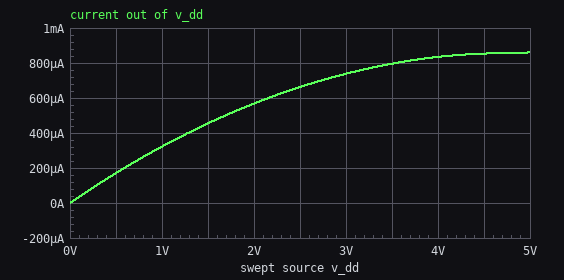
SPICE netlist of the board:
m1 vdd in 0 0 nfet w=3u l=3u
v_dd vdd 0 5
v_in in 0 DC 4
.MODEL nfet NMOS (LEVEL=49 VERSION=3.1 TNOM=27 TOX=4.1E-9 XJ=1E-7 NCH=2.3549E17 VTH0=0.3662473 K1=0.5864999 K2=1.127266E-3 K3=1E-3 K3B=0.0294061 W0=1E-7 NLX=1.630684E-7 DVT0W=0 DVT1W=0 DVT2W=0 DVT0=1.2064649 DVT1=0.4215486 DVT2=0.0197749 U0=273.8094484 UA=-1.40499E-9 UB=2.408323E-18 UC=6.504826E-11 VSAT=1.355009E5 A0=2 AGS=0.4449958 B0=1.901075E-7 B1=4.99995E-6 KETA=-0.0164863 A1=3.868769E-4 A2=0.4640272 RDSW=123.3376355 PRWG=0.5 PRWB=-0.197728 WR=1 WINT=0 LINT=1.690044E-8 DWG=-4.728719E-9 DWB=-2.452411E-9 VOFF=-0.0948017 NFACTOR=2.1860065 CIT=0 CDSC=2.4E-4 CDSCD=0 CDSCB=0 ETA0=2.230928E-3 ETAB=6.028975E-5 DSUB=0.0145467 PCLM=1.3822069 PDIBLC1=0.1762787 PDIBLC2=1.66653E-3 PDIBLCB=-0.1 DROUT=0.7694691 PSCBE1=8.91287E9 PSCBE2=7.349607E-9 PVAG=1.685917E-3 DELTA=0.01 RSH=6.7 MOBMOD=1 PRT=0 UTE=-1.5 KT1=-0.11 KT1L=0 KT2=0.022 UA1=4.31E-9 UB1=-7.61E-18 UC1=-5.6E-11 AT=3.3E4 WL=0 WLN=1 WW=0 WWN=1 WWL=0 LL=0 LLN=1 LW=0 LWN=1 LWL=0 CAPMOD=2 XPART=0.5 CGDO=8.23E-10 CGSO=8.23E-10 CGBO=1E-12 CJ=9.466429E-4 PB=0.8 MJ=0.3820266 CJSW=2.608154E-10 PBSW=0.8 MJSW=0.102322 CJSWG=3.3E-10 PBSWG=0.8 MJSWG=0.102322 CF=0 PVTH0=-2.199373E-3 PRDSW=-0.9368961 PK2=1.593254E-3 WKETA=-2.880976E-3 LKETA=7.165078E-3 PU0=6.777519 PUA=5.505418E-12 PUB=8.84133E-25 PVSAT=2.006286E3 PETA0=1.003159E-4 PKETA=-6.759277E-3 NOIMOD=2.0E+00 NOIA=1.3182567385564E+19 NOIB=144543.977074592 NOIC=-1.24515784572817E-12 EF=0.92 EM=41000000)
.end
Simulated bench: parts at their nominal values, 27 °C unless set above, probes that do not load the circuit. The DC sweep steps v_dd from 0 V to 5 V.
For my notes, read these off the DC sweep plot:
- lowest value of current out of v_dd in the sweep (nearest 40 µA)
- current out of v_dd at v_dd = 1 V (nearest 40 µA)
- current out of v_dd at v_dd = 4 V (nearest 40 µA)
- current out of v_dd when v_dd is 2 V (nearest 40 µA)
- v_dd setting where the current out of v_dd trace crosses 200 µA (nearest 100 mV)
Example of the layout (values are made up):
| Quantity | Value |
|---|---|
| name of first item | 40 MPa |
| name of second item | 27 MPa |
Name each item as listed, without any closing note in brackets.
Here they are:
| Quantity | Value |
|---|---|
| lowest value of current out of v_dd in the sweep | 0 A |
| current out of v_dd at v_dd = 1 V | 320 µA |
| current out of v_dd at v_dd = 4 V | 840 µA |
| current out of v_dd when v_dd is 2 V | 560 µA |
| v_dd setting where the current out of v_dd trace crosses 200 µA | 600 mV |
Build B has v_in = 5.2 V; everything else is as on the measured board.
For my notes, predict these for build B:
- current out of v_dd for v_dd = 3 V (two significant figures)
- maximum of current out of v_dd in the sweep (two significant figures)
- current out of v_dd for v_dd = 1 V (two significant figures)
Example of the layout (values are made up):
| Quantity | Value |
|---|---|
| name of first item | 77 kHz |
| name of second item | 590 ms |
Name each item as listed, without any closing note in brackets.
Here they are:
| Quantity | Value |
|---|---|
| current out of v_dd for v_dd = 3 V | 780 µA |
| maximum of current out of v_dd in the sweep | 1.1 mA |
| current out of v_dd for v_dd = 1 V | 290 µA |
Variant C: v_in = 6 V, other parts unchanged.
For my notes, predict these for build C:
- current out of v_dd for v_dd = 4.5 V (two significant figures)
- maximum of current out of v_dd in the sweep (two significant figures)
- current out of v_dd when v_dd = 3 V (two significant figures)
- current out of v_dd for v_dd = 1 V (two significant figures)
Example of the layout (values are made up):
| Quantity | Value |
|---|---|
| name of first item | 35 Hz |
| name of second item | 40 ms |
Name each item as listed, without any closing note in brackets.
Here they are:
| Quantity | Value |
|---|---|
| current out of v_dd for v_dd = 4.5 V | 1.1 mA |
| maximum of current out of v_dd in the sweep | 1.2 mA |
| current out of v_dd when v_dd = 3 V | 750 µA |
| current out of v_dd for v_dd = 1 V | 270 µA |
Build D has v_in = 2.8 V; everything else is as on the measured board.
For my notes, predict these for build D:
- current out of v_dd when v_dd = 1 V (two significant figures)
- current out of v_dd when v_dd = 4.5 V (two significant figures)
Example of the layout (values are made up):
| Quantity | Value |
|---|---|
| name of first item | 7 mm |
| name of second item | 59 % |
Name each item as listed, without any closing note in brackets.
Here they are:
| Quantity | Value |
|---|---|
| current out of v_dd when v_dd = 1 V | 310 µA |
| current out of v_dd when v_dd = 4.5 V | 470 µA |
